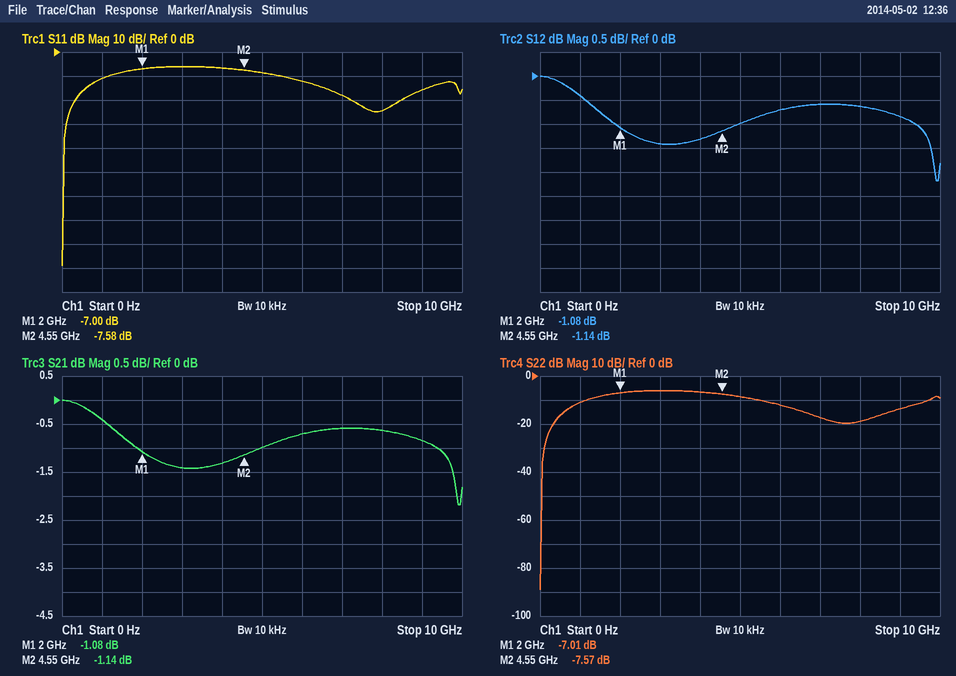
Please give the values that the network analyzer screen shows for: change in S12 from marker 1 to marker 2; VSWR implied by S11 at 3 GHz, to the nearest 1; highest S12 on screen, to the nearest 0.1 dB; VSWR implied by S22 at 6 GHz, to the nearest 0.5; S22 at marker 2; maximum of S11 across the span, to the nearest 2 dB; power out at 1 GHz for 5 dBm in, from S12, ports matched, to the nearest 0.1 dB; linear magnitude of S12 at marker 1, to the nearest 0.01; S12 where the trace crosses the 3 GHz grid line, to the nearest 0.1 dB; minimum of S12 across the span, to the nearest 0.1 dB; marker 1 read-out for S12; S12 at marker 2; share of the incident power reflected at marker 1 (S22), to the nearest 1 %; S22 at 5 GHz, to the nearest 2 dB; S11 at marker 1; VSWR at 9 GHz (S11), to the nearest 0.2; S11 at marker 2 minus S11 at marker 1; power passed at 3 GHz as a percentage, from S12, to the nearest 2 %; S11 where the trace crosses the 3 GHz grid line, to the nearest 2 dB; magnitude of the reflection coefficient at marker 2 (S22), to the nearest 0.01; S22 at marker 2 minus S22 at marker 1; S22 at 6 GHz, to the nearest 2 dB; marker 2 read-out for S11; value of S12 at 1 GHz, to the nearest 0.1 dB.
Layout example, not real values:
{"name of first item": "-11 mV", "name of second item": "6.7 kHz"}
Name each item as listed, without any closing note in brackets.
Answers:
{"change in S12 from marker 1 to marker 2": "-0.06 dB", "VSWR implied by S11 at 3 GHz, to the nearest 1": "3", "highest S12 on screen, to the nearest 0.1 dB": "0.0 dB", "VSWR implied by S22 at 6 GHz, to the nearest 0.5": "1.5", "S22 at marker 2": "-7.57 dB", "maximum of S11 across the span, to the nearest 2 dB": "-6 dB", "power out at 1 GHz for 5 dBm in, from S12, ports matched, to the nearest 0.1 dB": "4.6 dBm", "linear magnitude of S12 at marker 1, to the nearest 0.01": "0.88", "S12 where the trace crosses the 3 GHz grid line, to the nearest 0.1 dB": "-1.4 dB", "minimum of S12 across the span, to the nearest 0.1 dB": "-2.2 dB", "marker 1 read-out for S12": "-1.08 dB", "S12 at marker 2": "-1.14 dB", "share of the incident power reflected at marker 1 (S22), to the nearest 1 %": "20 %", "S22 at 5 GHz, to the nearest 2 dB": "-8 dB", "S11 at marker 1": "-7.00 dB", "VSWR at 9 GHz (S11), to the nearest 0.2": "1.4", "S11 at marker 2 minus S11 at marker 1": "-0.58 dB", "power passed at 3 GHz as a percentage, from S12, to the nearest 2 %": "72 %", "S11 where the trace crosses the 3 GHz grid line, to the nearest 2 dB": "-6 dB", "magnitude of the reflection coefficient at marker 2 (S22), to the nearest 0.01": "0.42", "S22 at marker 2 minus S22 at marker 1": "-0.56 dB", "S22 at 6 GHz, to the nearest 2 dB": "-12 dB", "marker 2 read-out for S11": "-7.58 dB", "value of S12 at 1 GHz, to the nearest 0.1 dB": "-0.4 dB"}
